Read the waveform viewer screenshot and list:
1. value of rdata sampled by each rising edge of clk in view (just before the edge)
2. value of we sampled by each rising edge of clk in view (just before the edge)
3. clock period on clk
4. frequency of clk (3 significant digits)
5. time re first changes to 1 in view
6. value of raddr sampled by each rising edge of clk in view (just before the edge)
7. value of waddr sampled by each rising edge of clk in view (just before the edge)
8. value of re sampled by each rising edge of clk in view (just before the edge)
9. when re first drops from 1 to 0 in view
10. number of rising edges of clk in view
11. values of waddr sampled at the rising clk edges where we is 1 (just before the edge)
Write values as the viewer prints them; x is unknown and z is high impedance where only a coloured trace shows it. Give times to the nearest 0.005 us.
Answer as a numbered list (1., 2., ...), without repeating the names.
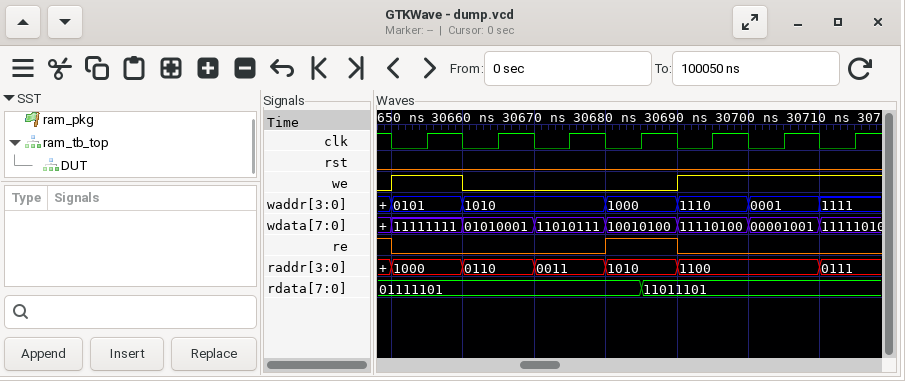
1. 01111101, 01111101, 01111101, 01111101, 11011101, 11011101, 11011101
2. 1 0 0 0 1 1 1
3. 0.01 us
4. 100 MHz
5. 30.68 us
6. 1000, 0110, 0011, 1010, 1100, 1100, 0111
7. 0101, 1010, 1010, 1000, 1110, 0001, 1111
8. 0 0 0 1 0 0 0
9. 30.65 us
10. 7
11. 0101, 1110, 0001, 1111
